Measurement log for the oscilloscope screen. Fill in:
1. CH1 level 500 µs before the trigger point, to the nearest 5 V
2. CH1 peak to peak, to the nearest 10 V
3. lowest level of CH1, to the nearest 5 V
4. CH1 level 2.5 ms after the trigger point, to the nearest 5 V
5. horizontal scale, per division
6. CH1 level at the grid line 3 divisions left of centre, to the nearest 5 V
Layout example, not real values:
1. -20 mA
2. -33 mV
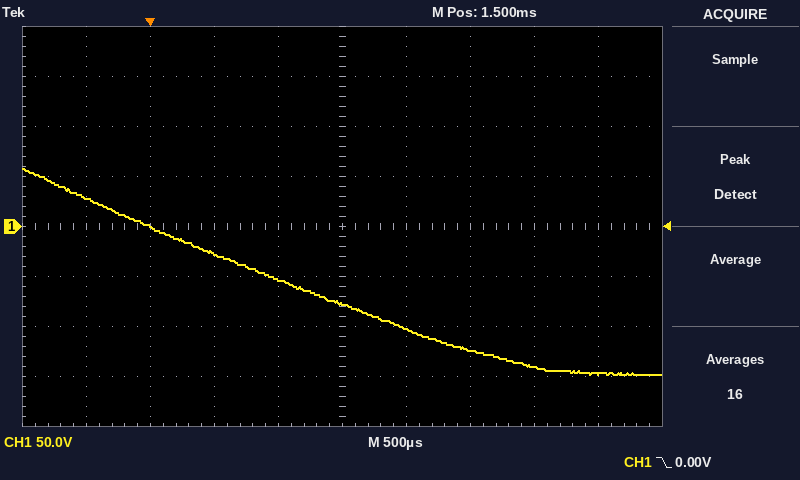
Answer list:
1. 30 V
2. 210 V
3. -150 V
4. -125 V
5. 500 µs
6. 0 V
